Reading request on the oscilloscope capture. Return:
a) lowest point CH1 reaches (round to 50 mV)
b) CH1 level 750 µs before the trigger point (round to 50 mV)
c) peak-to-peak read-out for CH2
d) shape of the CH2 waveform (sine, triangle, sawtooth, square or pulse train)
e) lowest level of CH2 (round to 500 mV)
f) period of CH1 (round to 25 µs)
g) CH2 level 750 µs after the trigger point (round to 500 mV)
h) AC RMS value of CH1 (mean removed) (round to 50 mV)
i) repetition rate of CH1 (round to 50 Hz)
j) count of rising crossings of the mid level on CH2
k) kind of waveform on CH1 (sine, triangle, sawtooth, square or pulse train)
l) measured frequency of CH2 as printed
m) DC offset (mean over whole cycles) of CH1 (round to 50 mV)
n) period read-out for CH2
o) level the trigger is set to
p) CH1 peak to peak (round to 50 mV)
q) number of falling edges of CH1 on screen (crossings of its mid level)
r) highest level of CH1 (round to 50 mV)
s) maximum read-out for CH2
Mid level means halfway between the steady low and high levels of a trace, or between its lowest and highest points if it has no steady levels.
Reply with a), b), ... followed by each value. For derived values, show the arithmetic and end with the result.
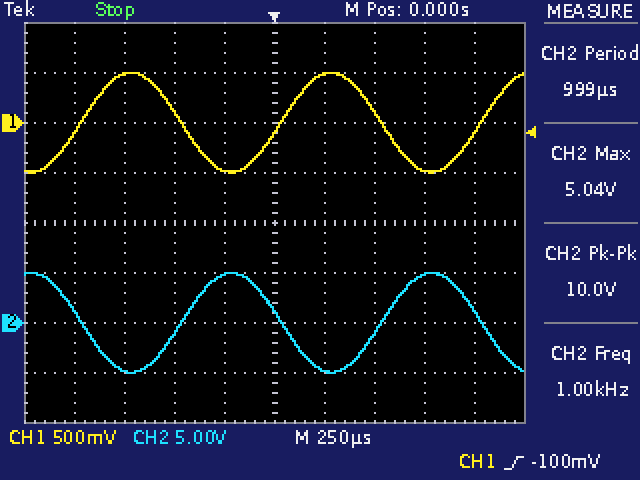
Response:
a) -500 mV
b) 500 mV
c) 10.0 V
d) sine
e) -5.0 V
f) 1.000 ms
g) 5.0 V
h) 1.00 V / (2√2) ≈ 354 mV, so 350 mV to the nearest 50 mV
i) 1 / 1.000 ms ≈ 1.00 kHz
j) 2
k) sine
l) 1.00 kHz
m) (500 mV + (-500 mV)) / 2 ≈ 0 mV
n) 999 µs
o) -100 mV
p) 500 mV − (-500 mV) = 1.00 V
q) 2
r) 500 mV
s) 5.04 V
